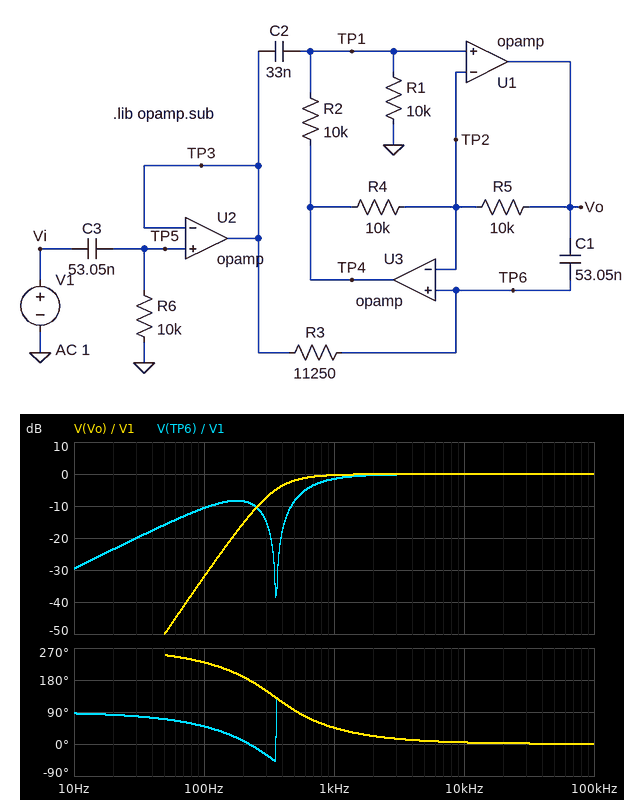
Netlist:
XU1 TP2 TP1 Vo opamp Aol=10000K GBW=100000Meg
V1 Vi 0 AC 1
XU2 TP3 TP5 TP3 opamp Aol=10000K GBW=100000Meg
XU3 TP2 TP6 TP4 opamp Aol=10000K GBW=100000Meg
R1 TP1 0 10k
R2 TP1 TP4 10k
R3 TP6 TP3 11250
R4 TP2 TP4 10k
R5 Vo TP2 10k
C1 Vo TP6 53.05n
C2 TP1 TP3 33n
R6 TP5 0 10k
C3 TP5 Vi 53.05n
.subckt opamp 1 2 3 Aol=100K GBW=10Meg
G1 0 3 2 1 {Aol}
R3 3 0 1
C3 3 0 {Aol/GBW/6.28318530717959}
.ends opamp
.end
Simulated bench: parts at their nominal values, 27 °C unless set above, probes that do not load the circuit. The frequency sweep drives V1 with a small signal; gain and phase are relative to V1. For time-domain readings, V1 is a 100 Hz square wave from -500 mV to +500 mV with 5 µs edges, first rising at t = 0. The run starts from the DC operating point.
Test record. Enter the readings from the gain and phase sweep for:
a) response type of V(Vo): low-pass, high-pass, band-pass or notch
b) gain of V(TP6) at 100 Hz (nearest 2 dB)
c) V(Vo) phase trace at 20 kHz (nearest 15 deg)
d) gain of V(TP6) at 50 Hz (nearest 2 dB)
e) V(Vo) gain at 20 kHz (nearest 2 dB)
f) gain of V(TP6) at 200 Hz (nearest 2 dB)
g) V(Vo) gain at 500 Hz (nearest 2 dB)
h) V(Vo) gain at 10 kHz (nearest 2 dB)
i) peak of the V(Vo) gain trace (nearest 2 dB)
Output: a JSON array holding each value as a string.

["high-pass", "-10 dB", "0 deg", "-16 dB", "0 dB", "-8 dB", "-2 dB", "0 dB", "0 dB"]
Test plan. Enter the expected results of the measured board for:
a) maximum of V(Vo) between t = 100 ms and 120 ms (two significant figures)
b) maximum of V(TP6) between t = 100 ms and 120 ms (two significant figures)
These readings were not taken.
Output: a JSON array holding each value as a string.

["990 mV", "990 mV"]
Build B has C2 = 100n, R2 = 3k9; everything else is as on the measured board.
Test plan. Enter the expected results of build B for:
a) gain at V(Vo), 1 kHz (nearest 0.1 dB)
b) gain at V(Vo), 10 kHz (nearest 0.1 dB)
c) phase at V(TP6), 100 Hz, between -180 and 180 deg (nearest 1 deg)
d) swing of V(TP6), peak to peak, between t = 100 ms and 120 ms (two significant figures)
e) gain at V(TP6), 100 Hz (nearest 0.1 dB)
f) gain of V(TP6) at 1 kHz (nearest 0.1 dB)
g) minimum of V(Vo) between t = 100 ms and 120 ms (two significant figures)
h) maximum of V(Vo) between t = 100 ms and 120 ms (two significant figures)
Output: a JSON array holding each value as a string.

["-0.1 dB", "0 dB", "62 deg", "1.9 V", "-10.1 dB", "-0.5 dB", "-960 mV", "960 mV"]
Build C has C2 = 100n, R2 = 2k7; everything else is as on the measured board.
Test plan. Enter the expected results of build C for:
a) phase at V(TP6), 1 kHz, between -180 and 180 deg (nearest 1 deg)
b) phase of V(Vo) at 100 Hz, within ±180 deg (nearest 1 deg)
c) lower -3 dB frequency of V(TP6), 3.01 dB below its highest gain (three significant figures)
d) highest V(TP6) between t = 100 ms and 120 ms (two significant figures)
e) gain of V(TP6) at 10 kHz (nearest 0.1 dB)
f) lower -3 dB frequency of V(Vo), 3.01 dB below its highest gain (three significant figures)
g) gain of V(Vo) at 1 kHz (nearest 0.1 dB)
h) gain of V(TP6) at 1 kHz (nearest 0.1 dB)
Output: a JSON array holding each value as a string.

["27 deg", "65 deg", "524 Hz", "1.0 V", "0 dB", "418 Hz", "-0.1 dB", "-0.5 dB"]
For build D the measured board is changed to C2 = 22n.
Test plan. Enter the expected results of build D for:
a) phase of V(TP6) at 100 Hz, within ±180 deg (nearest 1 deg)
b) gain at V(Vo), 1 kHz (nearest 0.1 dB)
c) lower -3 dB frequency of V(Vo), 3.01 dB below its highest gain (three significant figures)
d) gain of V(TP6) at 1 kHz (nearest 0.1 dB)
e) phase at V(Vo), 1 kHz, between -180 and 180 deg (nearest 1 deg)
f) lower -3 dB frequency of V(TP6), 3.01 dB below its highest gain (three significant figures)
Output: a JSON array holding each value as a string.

["50 deg", "-1.1 dB", "617 Hz", "-2.9 dB", "59 deg", "989 Hz"]
